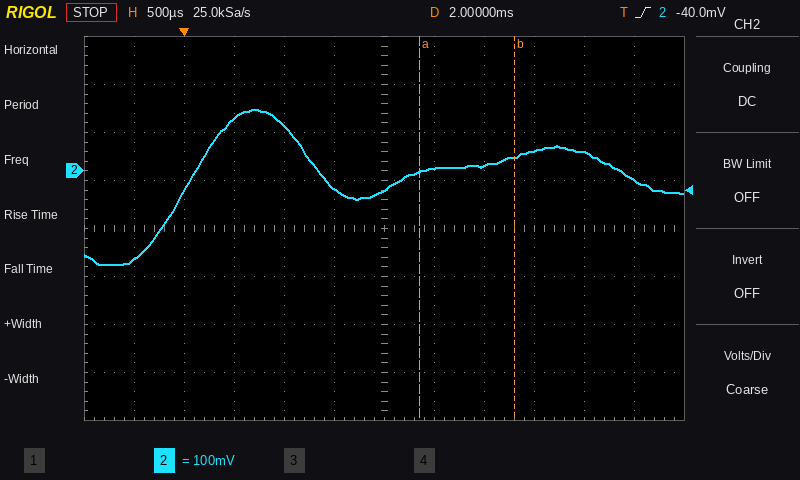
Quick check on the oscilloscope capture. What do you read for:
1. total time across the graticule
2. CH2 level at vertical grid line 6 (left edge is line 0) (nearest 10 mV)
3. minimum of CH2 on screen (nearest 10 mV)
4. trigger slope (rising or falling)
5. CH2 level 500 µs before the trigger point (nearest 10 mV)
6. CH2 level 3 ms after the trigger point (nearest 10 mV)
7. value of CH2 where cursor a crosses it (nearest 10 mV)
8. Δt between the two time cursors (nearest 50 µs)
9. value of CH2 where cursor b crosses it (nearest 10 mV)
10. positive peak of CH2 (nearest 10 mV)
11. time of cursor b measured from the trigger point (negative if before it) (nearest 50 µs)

6 ms
-40 mV
-200 mV
rising
-180 mV
10 mV
0 mV
950 µs
30 mV
130 mV
+3.30 ms
